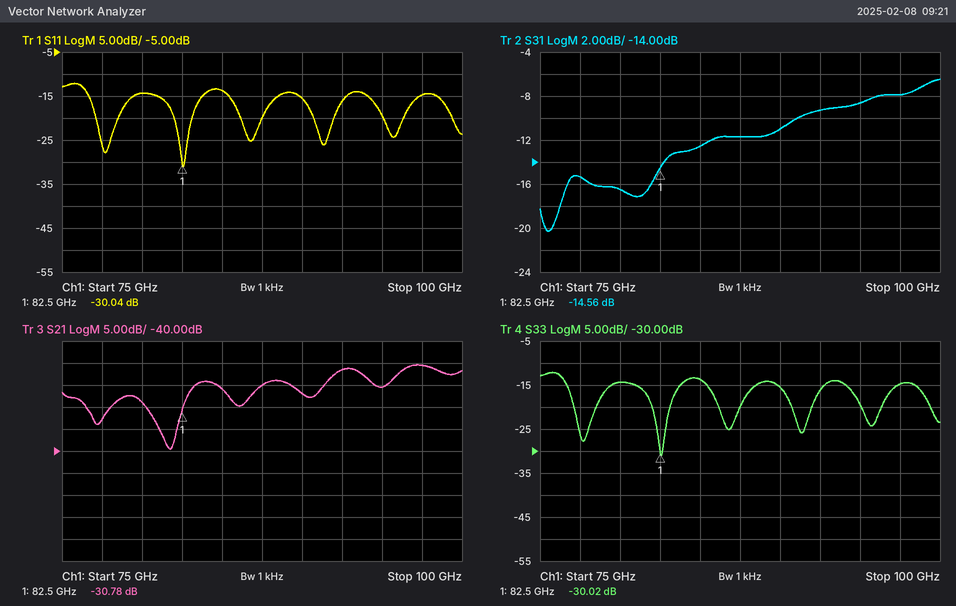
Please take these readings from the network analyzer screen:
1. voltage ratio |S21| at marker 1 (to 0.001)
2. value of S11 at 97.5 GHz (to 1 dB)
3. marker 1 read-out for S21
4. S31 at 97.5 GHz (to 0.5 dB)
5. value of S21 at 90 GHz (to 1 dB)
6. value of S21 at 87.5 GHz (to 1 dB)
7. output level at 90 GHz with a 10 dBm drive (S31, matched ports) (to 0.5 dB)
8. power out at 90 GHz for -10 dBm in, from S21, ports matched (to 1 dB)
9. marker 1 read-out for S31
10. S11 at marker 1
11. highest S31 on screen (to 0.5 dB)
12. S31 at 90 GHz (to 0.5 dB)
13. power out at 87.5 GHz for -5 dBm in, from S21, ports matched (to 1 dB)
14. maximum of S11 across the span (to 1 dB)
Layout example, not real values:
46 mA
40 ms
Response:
0.029
-15 dB
-30.78 dB
-8.0 dB
-27 dB
-25 dB
-1.0 dBm
-37 dBm
-14.56 dB
-30.04 dB
-6.5 dB
-11.0 dB
-30 dBm
-12 dB
